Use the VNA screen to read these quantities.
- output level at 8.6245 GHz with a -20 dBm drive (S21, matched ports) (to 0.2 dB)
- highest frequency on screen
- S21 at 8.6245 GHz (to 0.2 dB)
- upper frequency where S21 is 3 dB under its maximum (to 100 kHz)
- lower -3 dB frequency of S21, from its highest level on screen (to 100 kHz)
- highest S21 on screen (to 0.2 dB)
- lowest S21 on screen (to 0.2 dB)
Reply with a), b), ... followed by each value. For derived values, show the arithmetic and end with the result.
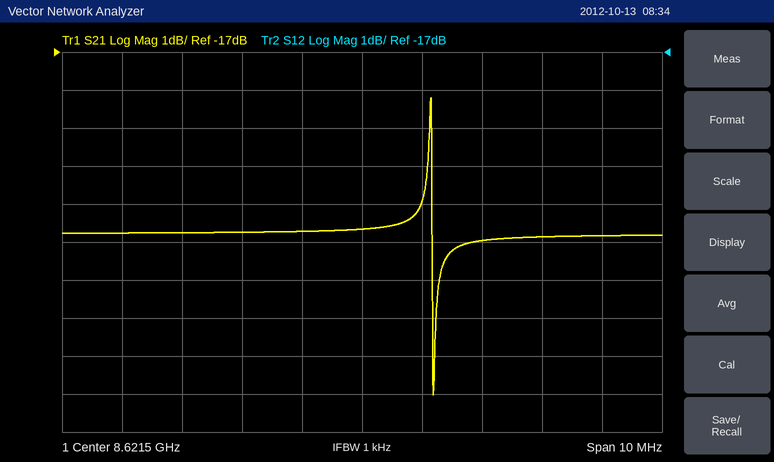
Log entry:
a) -20 dBm + (-21.8 dB) = -41.8 dBm
b) 8.6265 GHz
c) -21.8 dB
d) 8.6227 GHz
e) 8.6224 GHz
f) -18.2 dB
g) -26.0 dB
